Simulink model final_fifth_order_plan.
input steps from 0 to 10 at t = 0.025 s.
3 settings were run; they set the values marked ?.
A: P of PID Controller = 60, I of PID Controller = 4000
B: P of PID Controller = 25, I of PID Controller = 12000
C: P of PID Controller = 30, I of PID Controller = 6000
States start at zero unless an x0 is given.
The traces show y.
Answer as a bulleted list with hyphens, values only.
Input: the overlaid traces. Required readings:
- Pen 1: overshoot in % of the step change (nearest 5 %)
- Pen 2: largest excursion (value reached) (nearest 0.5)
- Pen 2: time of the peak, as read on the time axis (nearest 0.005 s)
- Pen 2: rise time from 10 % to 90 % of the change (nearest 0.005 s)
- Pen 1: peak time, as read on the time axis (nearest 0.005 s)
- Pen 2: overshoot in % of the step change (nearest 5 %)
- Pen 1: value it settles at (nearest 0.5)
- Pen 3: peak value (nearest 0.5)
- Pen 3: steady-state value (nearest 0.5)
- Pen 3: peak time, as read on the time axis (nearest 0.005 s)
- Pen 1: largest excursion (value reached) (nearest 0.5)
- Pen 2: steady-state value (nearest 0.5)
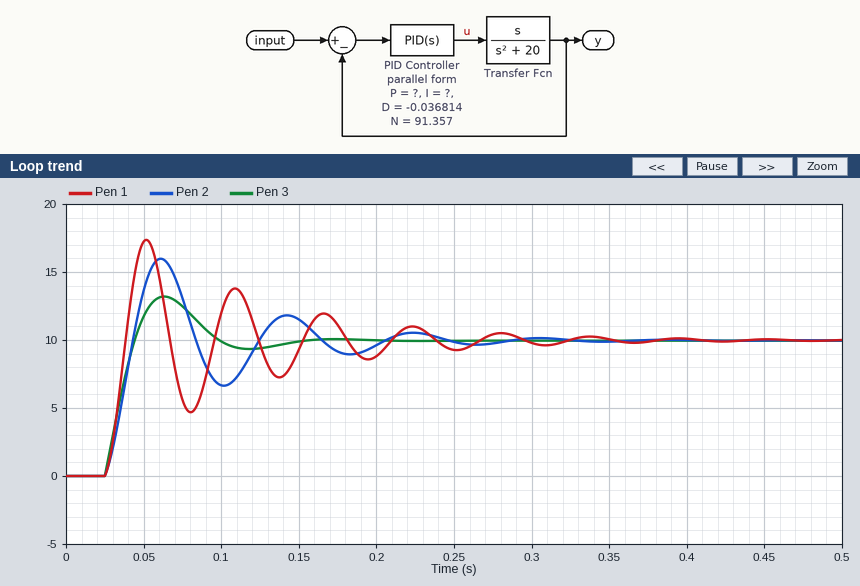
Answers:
- 75 %
- 16.0
- 0.060 s
- 0.015 s
- 0.050 s
- 60 %
- 10.0
- 13.0
- 10.0
- 0.065 s
- 17.5
- 10.0
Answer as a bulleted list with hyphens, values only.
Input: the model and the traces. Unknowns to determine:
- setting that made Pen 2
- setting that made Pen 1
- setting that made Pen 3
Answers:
- C
- B
- A
